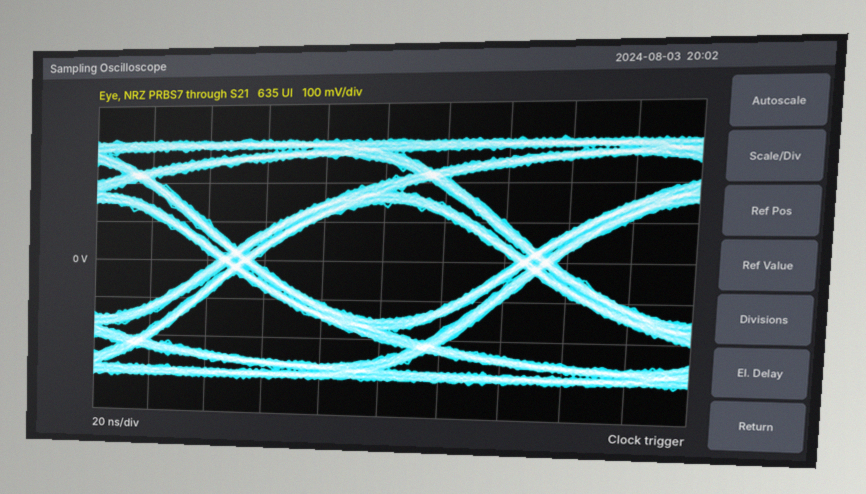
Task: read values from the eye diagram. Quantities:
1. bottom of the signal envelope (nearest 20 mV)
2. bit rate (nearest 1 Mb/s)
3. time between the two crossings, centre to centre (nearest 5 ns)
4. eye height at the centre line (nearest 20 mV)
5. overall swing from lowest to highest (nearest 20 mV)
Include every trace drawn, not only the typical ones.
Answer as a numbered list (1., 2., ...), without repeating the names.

1. -320 mV
2. 10 Mb/s
3. 100 ns
4. 300 mV
5. 620 mV
